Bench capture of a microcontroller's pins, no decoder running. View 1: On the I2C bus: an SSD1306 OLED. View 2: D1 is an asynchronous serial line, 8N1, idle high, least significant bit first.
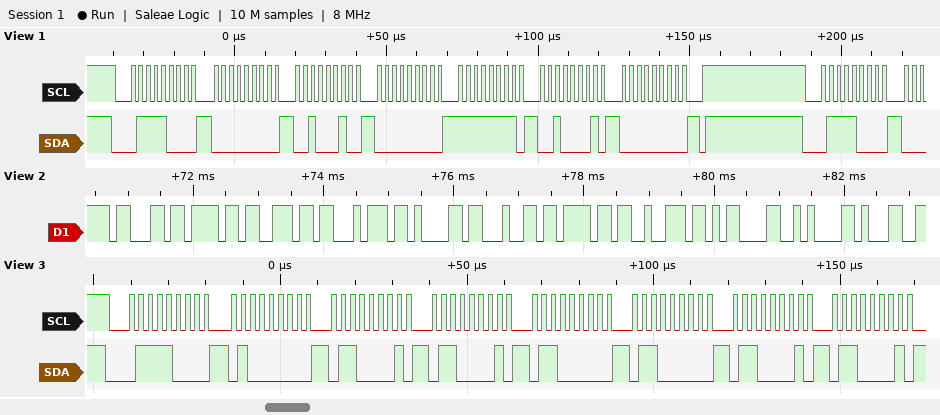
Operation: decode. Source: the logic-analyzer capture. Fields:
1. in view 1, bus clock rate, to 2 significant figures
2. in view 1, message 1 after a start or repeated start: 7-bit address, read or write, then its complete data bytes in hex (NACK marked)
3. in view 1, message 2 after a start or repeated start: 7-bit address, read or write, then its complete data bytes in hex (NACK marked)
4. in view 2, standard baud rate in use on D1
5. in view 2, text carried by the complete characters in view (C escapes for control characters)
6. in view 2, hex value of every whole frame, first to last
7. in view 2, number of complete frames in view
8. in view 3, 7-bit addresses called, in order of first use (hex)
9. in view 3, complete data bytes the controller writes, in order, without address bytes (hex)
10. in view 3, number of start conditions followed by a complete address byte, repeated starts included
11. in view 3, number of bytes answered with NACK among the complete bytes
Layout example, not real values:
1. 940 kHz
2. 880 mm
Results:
1. 400 kHz
2. 0x3C write: 00 22 00 FF 21 00
3. 0x3C write
4. 9600 baud
5. "contador\r\n1"
6. 63 6F 6E 74 61 64 6F 72 0D 0A 31
7. 11
8. 0x3C
9. 40 61 61 60 60 61 61
10. 1
11. 0
